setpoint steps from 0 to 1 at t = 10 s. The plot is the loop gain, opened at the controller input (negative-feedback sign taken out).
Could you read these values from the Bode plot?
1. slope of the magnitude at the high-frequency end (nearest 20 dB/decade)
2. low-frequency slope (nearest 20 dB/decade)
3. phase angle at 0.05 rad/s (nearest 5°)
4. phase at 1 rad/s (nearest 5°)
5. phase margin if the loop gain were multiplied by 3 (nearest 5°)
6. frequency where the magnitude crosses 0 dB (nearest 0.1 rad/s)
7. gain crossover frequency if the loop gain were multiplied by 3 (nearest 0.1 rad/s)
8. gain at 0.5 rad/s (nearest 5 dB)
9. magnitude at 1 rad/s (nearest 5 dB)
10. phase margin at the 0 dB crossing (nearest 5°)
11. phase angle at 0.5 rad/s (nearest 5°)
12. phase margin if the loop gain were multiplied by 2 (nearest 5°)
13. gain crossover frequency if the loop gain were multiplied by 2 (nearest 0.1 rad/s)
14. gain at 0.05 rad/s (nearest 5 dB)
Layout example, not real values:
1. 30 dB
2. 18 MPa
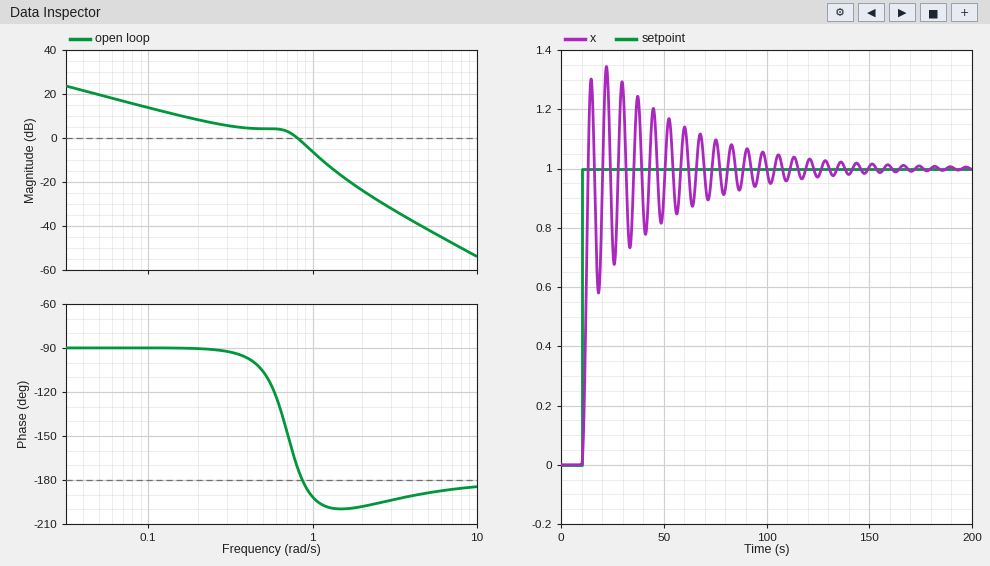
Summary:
1. -40 dB/decade
2. -20 dB/decade
3. -90°
4. -190°
5. -15°
6. 0.8 rad/s
7. 1.1 rad/s
8. 5 dB
9. -5 dB
10. 10°
11. -105°
12. -10°
13. 1.0 rad/s
14. 20 dB
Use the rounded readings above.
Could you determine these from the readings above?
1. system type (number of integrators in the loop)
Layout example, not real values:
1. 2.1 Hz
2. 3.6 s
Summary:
1. 1
